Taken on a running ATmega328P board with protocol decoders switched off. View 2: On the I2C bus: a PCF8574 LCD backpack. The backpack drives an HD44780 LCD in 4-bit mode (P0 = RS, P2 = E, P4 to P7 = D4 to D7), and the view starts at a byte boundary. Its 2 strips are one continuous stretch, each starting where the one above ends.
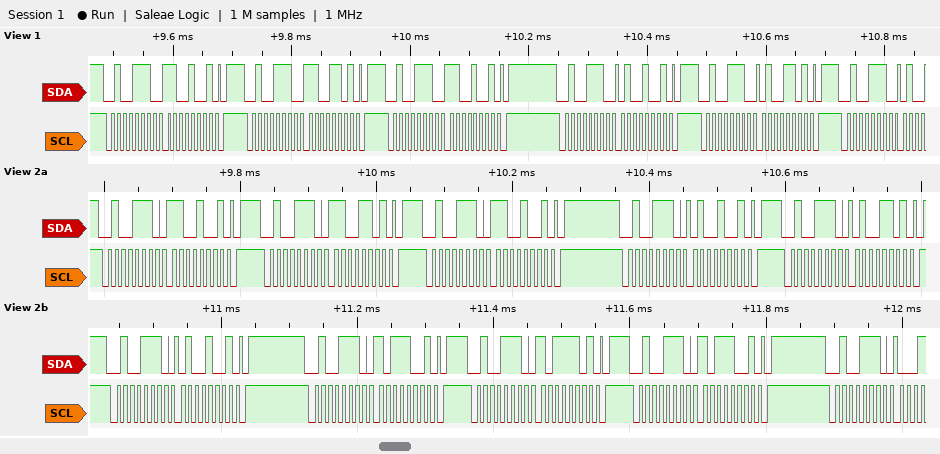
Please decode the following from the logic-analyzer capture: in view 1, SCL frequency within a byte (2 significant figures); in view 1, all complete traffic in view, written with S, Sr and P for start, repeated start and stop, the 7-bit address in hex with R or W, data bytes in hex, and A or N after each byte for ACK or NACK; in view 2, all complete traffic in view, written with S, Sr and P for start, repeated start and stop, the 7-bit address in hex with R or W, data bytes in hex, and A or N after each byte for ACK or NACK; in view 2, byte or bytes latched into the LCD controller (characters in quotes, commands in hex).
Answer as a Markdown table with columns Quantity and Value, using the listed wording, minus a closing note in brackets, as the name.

| Quantity | Value |
|---|---|
| in view 1, SCL frequency within a byte | 100 kHz |
| in view 1, all complete traffic in view, written with S, Sr and P for start, repeated start and stop, the 7-bit address in hex with R or W, data bytes in hex, and A or N after each byte for ACK or NACK | S 27W A C9 A P S 27W A CD A P S 27W A C9 A P S 27W A 49 A P S 27W A 4D A P S 27W A |
| in view 2, all complete traffic in view, written with S, Sr and P for start, repeated start and stop, the 7-bit address in hex with R or W, data bytes in hex, and A or N after each byte for ACK or NACK | S 27W A C9 A P S 27W A CD A P S 27W A C9 A P S 27W A 49 A P S 27W A 4D A P S 27W A 49 A P S 27W A B9 A P S 27W A BD A P S 27W A B9 A P S 27W A |
| in view 2, byte or bytes latched into the LCD controller | data 0xC4 |
